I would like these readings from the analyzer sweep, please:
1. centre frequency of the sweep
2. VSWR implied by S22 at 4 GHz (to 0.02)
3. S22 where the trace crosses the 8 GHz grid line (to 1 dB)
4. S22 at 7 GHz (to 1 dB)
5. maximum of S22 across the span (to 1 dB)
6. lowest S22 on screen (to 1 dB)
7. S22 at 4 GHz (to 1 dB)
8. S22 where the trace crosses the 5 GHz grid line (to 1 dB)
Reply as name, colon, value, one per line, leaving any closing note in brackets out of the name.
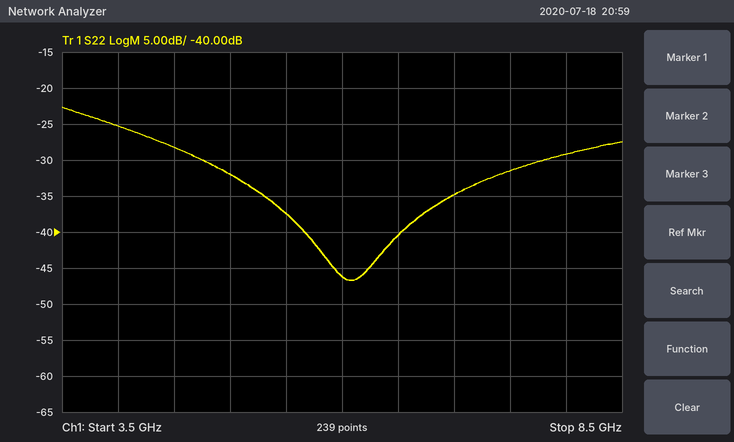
centre frequency of the sweep: 6 GHz
VSWR implied by S22 at 4 GHz: 1.12
S22 where the trace crosses the 8 GHz grid line: -29 dB
S22 at 7 GHz: -35 dB
maximum of S22 across the span: -23 dB
lowest S22 on screen: -47 dB
S22 at 4 GHz: -25 dB
S22 where the trace crosses the 5 GHz grid line: -32 dB
